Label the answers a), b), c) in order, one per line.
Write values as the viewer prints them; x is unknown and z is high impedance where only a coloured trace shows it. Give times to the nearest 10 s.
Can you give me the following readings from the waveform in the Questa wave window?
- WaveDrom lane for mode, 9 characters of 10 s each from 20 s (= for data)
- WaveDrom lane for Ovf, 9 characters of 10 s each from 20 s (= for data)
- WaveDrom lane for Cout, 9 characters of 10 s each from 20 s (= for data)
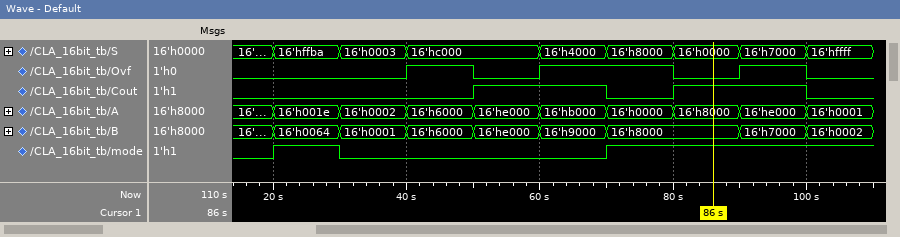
a) {name: 'mode', wave: '10...1...'}
b) {name: 'Ovf', wave: '0.101.010'}
c) {name: 'Cout', wave: '0..1.01.0'}
